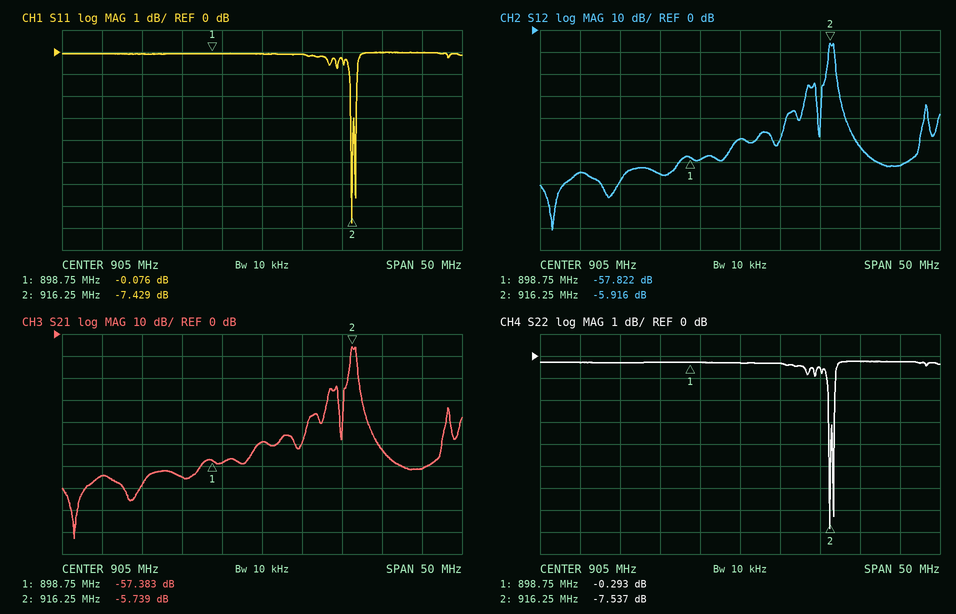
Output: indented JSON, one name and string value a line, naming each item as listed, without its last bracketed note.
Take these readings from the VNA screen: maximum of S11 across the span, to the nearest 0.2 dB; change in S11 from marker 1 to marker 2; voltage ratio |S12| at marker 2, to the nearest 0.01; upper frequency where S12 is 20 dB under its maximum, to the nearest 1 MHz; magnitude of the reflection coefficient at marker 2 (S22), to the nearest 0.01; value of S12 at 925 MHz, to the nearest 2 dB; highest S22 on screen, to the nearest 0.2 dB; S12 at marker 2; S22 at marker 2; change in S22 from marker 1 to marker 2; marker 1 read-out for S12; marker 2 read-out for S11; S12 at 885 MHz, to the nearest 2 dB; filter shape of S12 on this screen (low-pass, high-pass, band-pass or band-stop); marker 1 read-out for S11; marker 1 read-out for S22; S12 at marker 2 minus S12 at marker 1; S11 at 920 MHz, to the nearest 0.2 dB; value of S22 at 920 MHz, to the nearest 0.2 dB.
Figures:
{
  "maximum of S11 across the span, to the nearest 0.2 dB": "0.0 dB",
  "change in S11 from marker 1 to marker 2": "-7.353 dB",
  "voltage ratio |S12| at marker 2, to the nearest 0.01": "0.51",
  "upper frequency where S12 is 20 dB under its maximum, to the nearest 1 MHz": "917 MHz",
  "magnitude of the reflection coefficient at marker 2 (S22), to the nearest 0.01": "0.42",
  "value of S12 at 925 MHz, to the nearest 2 dB": "-62 dB",
  "highest S22 on screen, to the nearest 0.2 dB": "-0.2 dB",
  "S12 at marker 2": "-5.916 dB",
  "S22 at marker 2": "-7.537 dB",
  "change in S22 from marker 1 to marker 2": "-7.244 dB",
  "marker 1 read-out for S12": "-57.822 dB",
  "marker 2 read-out for S11": "-7.429 dB",
  "S12 at 885 MHz, to the nearest 2 dB": "-64 dB",
  "filter shape of S12 on this screen": "band-pass",
  "marker 1 read-out for S11": "-0.076 dB",
  "marker 1 read-out for S22": "-0.293 dB",
  "S12 at marker 2 minus S12 at marker 1": "51.906 dB",
  "S11 at 920 MHz, to the nearest 0.2 dB": "0.0 dB",
  "value of S22 at 920 MHz, to the nearest 0.2 dB": "-0.2 dB"
}
